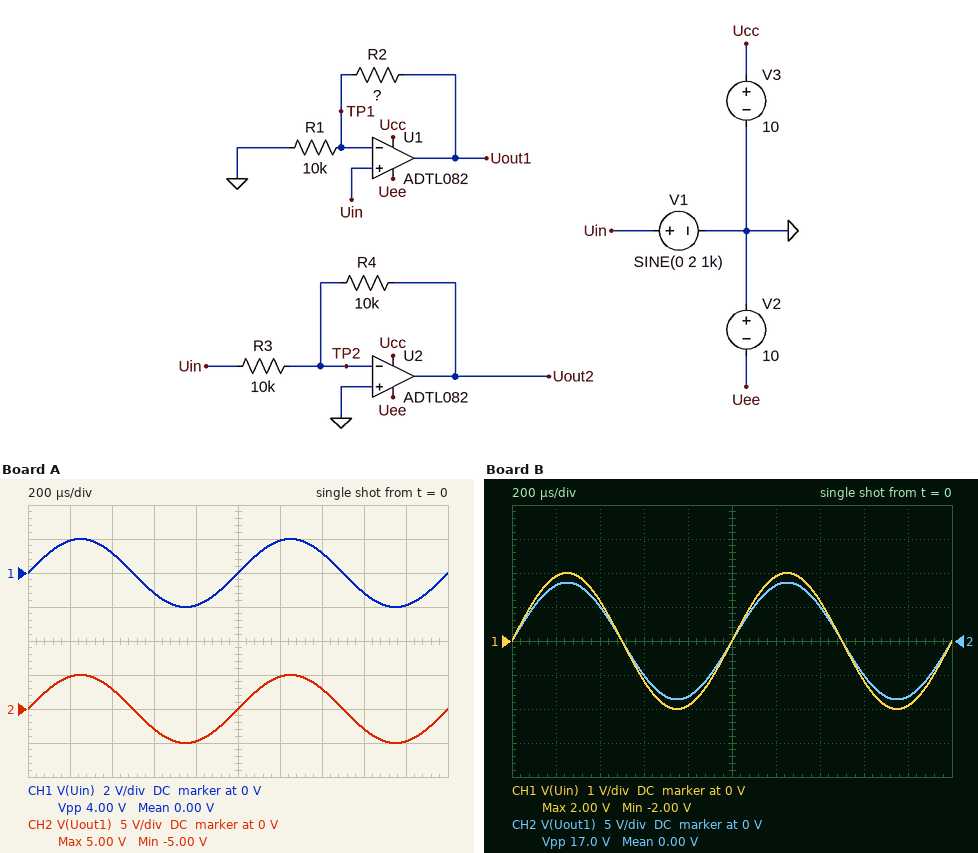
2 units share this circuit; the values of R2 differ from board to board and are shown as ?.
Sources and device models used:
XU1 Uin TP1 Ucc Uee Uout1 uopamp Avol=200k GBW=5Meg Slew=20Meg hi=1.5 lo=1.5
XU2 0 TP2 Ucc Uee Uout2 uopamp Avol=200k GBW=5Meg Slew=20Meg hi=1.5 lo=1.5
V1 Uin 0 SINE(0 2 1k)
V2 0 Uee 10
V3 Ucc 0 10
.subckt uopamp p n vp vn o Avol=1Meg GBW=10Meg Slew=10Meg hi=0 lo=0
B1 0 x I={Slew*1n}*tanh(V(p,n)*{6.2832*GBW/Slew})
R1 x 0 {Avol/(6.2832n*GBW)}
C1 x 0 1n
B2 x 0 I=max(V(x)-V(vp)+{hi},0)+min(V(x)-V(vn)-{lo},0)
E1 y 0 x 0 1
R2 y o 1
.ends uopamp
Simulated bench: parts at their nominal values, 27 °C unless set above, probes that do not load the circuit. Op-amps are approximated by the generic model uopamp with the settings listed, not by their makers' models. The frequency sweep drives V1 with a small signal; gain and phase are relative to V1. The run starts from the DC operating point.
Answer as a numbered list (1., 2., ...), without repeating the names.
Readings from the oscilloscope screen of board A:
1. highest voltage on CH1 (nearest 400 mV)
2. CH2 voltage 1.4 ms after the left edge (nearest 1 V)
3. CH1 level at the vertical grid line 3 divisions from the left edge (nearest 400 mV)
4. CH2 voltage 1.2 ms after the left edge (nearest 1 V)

1. 2.0 V
2. 3 V
3. -1.2 V
4. 5 V
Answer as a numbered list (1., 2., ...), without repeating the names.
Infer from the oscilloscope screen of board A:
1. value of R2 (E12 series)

1. 15 kΩ
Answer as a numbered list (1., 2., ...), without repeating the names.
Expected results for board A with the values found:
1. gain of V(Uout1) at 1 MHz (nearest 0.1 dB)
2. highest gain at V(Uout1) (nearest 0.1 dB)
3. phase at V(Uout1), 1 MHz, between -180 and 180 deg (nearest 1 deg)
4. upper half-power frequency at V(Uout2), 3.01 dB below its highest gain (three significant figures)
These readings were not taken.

1. 7.0 dB
2. 8.0 dB
3. -27 deg
4. 2.50 MHz
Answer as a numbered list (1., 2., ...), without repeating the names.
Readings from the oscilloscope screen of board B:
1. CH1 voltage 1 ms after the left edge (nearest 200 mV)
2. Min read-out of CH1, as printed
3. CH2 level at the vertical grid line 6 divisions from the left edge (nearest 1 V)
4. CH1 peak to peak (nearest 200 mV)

1. 0 V
2. -2.00 V
3. 8 V
4. 4.0 V
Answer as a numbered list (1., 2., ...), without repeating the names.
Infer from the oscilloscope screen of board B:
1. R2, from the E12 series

1. 33 kΩ
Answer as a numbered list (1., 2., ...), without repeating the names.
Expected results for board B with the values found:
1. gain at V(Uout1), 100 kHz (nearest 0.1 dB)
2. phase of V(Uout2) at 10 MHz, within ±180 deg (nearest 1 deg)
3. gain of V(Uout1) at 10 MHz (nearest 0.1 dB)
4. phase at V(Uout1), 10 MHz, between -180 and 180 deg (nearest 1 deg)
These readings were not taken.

1. 12.6 dB
2. 104 deg
3. -6.1 dB
4. -83 deg
